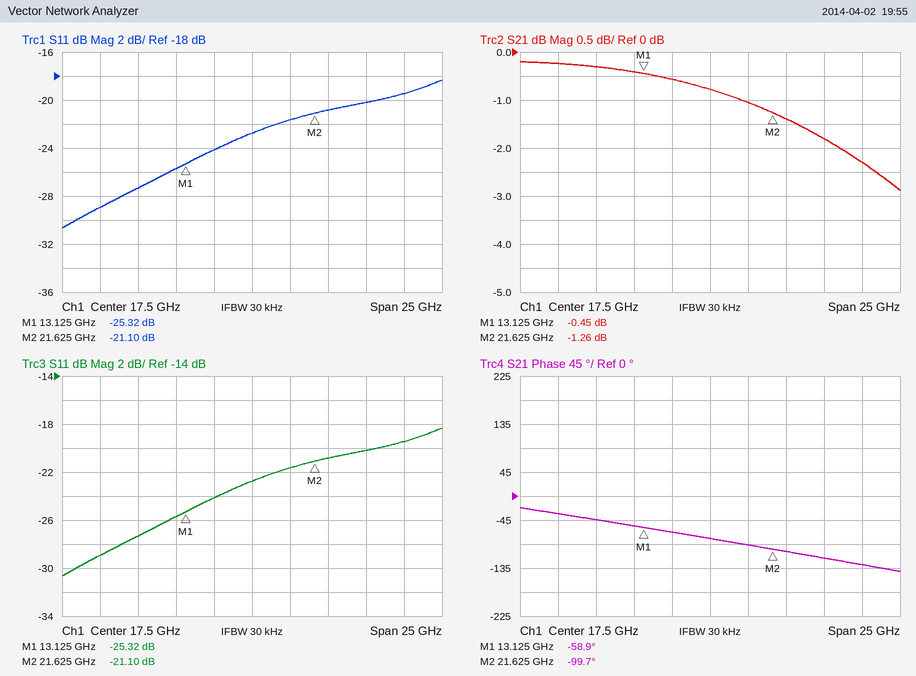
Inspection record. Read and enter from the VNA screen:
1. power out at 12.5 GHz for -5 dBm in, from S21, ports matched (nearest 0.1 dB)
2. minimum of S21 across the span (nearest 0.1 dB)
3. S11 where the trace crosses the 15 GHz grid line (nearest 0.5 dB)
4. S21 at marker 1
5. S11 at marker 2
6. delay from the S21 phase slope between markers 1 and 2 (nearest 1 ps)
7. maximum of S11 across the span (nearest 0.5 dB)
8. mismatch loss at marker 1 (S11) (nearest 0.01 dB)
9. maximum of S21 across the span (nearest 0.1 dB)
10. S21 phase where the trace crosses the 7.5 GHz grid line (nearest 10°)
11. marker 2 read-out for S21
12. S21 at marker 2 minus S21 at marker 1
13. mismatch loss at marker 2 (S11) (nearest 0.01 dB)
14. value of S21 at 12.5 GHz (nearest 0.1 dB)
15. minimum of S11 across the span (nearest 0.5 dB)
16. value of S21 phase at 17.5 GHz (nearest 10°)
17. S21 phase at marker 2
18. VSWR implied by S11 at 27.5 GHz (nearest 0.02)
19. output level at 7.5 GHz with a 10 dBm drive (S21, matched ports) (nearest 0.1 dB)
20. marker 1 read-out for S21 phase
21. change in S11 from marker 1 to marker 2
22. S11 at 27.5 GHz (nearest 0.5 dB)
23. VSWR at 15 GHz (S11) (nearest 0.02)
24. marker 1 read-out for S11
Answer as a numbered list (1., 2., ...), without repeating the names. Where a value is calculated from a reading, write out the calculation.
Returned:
1. -5 dBm + (-0.4 dB) = -5.4 dBm
2. -2.9 dB
3. -24.0 dB
4. -0.45 dB
5. -21.10 dB
6. −(-99.7° − (-58.9°))/(360° × 8.5 GHz) ≈ 13 ps
7. -18.5 dB
8. −10 log10(1 − 10^(-25.32/10)) ≈ 0.01 dB
9. -0.2 dB
10. -30°
11. -1.26 dB
12. -1.26 − (-0.45) = -0.81 dB
13. −10 log10(1 − 10^(-21.1/10)) ≈ 0.03 dB
14. -0.4 dB
15. -30.5 dB
16. -80°
17. -99.7°
18. |Γ| = 10^(-19.5/20) = 0.1059; VSWR = (1 + 0.1059)/(1 − 0.1059) ≈ 1.24
19. 10 dBm + (-0.2 dB) = 9.8 dBm
20. -58.9°
21. -21.1 − (-25.32) = 4.22 dB
22. -19.5 dB
23. |Γ| = 10^(-24/20) = 0.0631; VSWR = (1 + 0.0631)/(1 − 0.0631) ≈ 1.13, so 1.14 to the nearest 0.02
24. -25.32 dB
